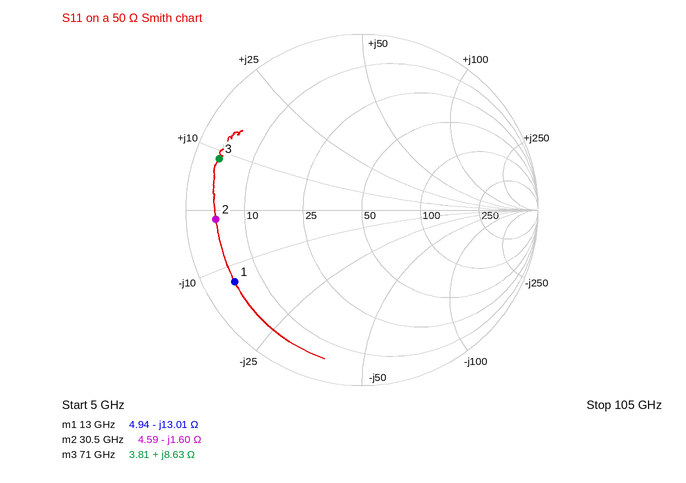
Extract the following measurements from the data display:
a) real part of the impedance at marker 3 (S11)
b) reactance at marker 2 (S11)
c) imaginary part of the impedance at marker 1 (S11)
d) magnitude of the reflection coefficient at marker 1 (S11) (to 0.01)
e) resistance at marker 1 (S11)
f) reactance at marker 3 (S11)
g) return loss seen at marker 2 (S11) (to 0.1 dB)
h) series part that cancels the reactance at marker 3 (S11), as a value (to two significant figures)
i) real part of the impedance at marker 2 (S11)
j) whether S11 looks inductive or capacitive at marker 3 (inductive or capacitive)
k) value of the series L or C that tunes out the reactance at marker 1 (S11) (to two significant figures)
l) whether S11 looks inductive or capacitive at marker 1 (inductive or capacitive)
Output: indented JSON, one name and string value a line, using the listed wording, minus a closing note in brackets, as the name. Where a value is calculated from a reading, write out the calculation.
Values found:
{
  "real part of the impedance at marker 3": "3.81 Ω",
  "reactance at marker 2": "-1.60 Ω",
  "imaginary part of the impedance at marker 1": "-13.01 Ω",
  "magnitude of the reflection coefficient at marker 1 (S11)": "0.83",
  "resistance at marker 1": "4.94 Ω",
  "reactance at marker 3": "+8.63 Ω",
  "return loss seen at marker 2 (S11)": "1.6 dB",
  "series part that cancels the reactance at marker 3 (S11), as a value": "C = 1/(2π × 71 GHz × 8.63 Ω) ≈ 260 fF",
  "real part of the impedance at marker 2": "4.59 Ω",
  "whether S11 looks inductive or capacitive at marker 3": "inductive",
  "value of the series L or C that tunes out the reactance at marker 1 (S11)": "L = 13.01 Ω/(2π × 13 GHz) ≈ 159 pH, so 160 pH to two significant figures",
  "whether S11 looks inductive or capacitive at marker 1": "capacitive"
}
